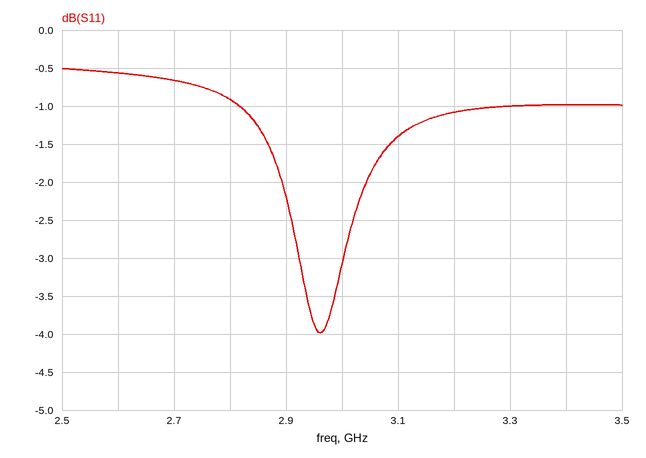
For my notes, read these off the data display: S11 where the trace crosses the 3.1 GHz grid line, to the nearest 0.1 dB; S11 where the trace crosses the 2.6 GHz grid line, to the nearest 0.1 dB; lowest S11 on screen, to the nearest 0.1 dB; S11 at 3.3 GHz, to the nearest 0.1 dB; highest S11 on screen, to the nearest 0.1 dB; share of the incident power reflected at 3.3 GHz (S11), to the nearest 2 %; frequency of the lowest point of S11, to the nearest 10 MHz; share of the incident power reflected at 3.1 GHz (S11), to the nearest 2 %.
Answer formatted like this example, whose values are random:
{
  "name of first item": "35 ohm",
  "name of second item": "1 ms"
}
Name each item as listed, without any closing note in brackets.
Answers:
{
  "S11 where the trace crosses the 3.1 GHz grid line, to the nearest 0.1 dB": "-1.4 dB",
  "S11 where the trace crosses the 2.6 GHz grid line, to the nearest 0.1 dB": "-0.6 dB",
  "lowest S11 on screen, to the nearest 0.1 dB": "-4.0 dB",
  "S11 at 3.3 GHz, to the nearest 0.1 dB": "-1.0 dB",
  "highest S11 on screen, to the nearest 0.1 dB": "-0.5 dB",
  "share of the incident power reflected at 3.3 GHz (S11), to the nearest 2 %": "80 %",
  "frequency of the lowest point of S11, to the nearest 10 MHz": "2.96 GHz",
  "share of the incident power reflected at 3.1 GHz (S11), to the nearest 2 %": "72 %"
}
